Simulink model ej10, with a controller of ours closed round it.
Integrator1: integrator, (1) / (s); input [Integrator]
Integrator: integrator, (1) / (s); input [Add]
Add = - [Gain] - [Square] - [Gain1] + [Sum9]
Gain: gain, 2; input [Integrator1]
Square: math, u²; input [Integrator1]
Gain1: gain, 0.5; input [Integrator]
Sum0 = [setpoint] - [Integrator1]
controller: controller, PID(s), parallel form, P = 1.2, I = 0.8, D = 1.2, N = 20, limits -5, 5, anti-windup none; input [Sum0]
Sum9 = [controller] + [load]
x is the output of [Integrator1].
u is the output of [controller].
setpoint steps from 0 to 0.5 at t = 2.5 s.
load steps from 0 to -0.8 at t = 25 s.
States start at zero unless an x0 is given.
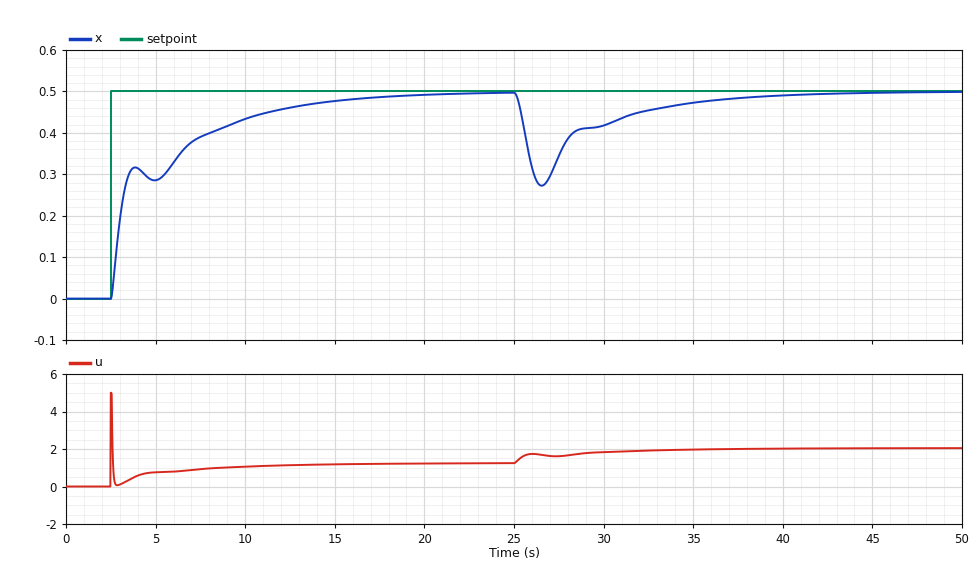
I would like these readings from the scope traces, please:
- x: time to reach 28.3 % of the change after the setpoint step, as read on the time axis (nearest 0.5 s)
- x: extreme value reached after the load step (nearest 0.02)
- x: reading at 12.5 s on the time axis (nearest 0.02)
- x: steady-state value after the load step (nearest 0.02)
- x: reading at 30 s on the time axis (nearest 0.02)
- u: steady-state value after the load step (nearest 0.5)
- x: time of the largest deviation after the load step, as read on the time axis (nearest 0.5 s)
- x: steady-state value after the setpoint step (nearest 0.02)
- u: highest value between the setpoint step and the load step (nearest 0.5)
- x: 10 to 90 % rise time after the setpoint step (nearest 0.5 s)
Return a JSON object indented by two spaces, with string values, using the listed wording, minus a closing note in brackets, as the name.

{
  "x: time to reach 28.3 % of the change after the setpoint step, as read on the time axis": "3.0 s",
  "x: extreme value reached after the load step": "0.28",
  "x: reading at 12.5 s on the time axis": "0.46",
  "x: steady-state value after the load step": "0.50",
  "x: reading at 30 s on the time axis": "0.42",
  "u: steady-state value after the load step": "2.0",
  "x: time of the largest deviation after the load step, as read on the time axis": "26.5 s",
  "x: steady-state value after the setpoint step": "0.50",
  "u: highest value between the setpoint step and the load step": "5.0",
  "x: 10 to 90 % rise time after the setpoint step": "8.5 s"
}
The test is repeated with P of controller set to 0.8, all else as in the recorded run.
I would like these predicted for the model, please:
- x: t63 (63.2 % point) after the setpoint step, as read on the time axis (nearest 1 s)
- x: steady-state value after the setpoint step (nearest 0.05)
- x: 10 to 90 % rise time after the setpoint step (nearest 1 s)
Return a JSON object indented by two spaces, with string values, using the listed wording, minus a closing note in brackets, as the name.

{
  "x: t63 (63.2 % point) after the setpoint step, as read on the time axis": "6 s",
  "x: steady-state value after the setpoint step": "0.50",
  "x: 10 to 90 % rise time after the setpoint step": "8 s"
}
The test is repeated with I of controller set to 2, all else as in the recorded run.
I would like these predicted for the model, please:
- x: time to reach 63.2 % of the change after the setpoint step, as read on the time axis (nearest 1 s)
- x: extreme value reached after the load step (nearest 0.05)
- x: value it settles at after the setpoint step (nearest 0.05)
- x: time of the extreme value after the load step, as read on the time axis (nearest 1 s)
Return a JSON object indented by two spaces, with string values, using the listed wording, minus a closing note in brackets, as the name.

{
  "x: time to reach 63.2 % of the change after the setpoint step, as read on the time axis": "3 s",
  "x: extreme value reached after the load step": "0.30",
  "x: value it settles at after the setpoint step": "0.50",
  "x: time of the extreme value after the load step, as read on the time axis": "26 s"
}
